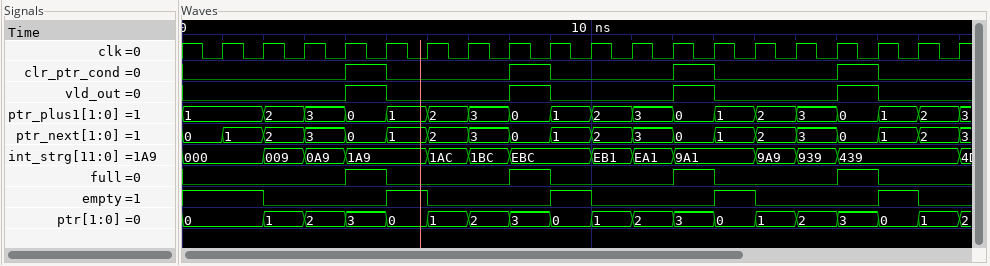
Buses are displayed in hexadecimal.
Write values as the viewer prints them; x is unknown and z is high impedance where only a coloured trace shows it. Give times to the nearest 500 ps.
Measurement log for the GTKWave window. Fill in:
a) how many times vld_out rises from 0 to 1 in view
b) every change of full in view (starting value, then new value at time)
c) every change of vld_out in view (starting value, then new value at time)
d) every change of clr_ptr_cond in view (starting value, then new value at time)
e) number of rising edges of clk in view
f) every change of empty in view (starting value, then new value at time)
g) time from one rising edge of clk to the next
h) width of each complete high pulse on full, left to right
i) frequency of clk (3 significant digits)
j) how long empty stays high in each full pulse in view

4
0, 1 at 4000 ps, 0 at 5000 ps, 1 at 8000 ps, 0 at 9000 ps, 1 at 12000 ps, 0 at 13000 ps, 1 at 16000 ps, 0 at 17000 ps
0, 1 at 4000 ps, 0 at 5000 ps, 1 at 8000 ps, 0 at 9000 ps, 1 at 12000 ps, 0 at 13000 ps, 1 at 16000 ps, 0 at 17000 ps
0, 1 at 4000 ps, 0 at 5000 ps, 1 at 8000 ps, 0 at 9000 ps, 1 at 12000 ps, 0 at 13000 ps, 1 at 16000 ps, 0 at 17000 ps
19
1, 0 at 2000 ps, 1 at 5000 ps, 0 at 6000 ps, 1 at 9000 ps, 0 at 10000 ps, 1 at 13000 ps, 0 at 14000 ps, 1 at 17000 ps, 0 at 18000 ps
1000 ps
1000 ps, 1000 ps, 1000 ps, 1000 ps
1.00 GHz
1000 ps, 1000 ps, 1000 ps, 1000 ps
